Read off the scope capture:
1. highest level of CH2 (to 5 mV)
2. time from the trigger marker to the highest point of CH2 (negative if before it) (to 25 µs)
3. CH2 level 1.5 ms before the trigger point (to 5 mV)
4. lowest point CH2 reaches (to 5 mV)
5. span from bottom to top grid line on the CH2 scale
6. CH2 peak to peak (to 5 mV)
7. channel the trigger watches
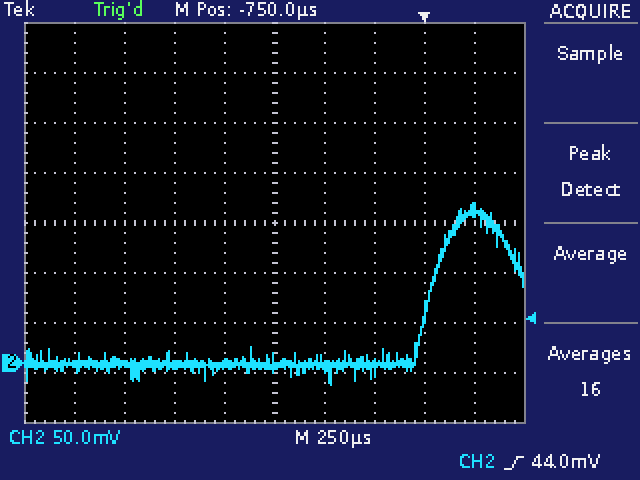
160 mV
+250 µs
0 mV
-20 mV
400 mV
180 mV
CH2
